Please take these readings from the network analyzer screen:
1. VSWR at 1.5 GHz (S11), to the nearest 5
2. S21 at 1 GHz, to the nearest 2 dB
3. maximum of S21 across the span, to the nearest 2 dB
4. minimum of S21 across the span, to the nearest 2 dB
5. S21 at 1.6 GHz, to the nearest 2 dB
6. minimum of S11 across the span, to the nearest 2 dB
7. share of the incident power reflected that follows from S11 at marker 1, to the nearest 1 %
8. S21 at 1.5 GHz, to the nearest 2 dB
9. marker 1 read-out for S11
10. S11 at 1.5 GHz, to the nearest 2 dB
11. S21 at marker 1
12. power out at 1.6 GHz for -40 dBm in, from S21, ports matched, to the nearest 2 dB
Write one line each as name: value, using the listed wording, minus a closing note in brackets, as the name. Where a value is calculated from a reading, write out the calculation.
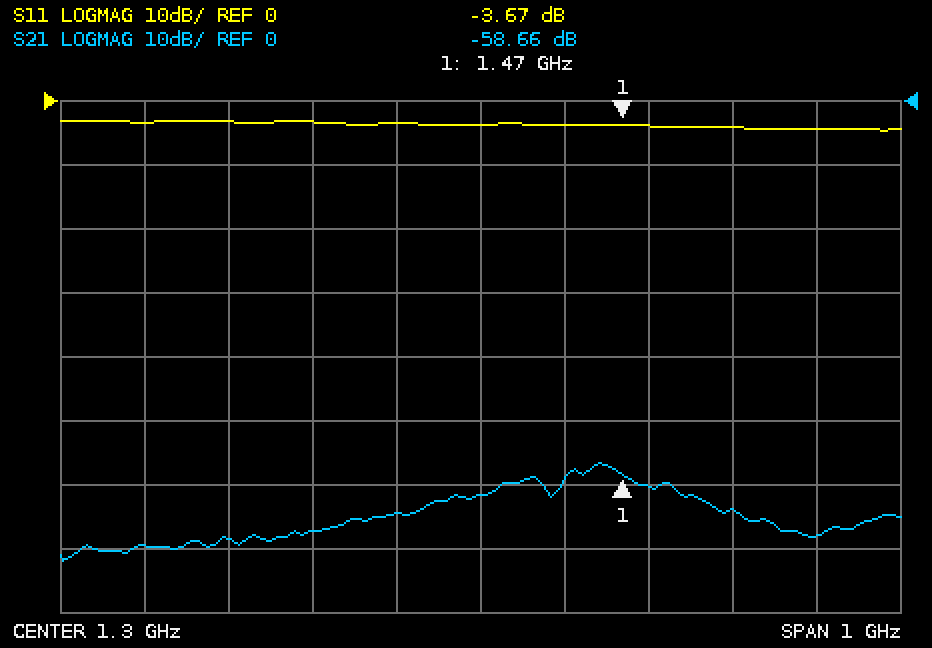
VSWR at 1.5 GHz (S11), to the nearest 5: |Γ| = 10^(-4/20) = 0.6310; VSWR = (1 + 0.6310)/(1 − 0.6310) ≈ 4.42, so 5 to the nearest 5
S21 at 1 GHz, to the nearest 2 dB: -68 dB
maximum of S21 across the span, to the nearest 2 dB: -56 dB
minimum of S21 across the span, to the nearest 2 dB: -72 dB
S21 at 1.6 GHz, to the nearest 2 dB: -64 dB
minimum of S11 across the span, to the nearest 2 dB: -4 dB
share of the incident power reflected that follows from S11 at marker 1, to the nearest 1 %: 10^(-3.67/10) ≈ 43 %
S21 at 1.5 GHz, to the nearest 2 dB: -60 dB
marker 1 read-out for S11: -3.67 dB
S11 at 1.5 GHz, to the nearest 2 dB: -4 dB
S21 at marker 1: -58.66 dB
power out at 1.6 GHz for -40 dBm in, from S21, ports matched, to the nearest 2 dB: -40 dBm + (-64 dB) = -104 dBm
